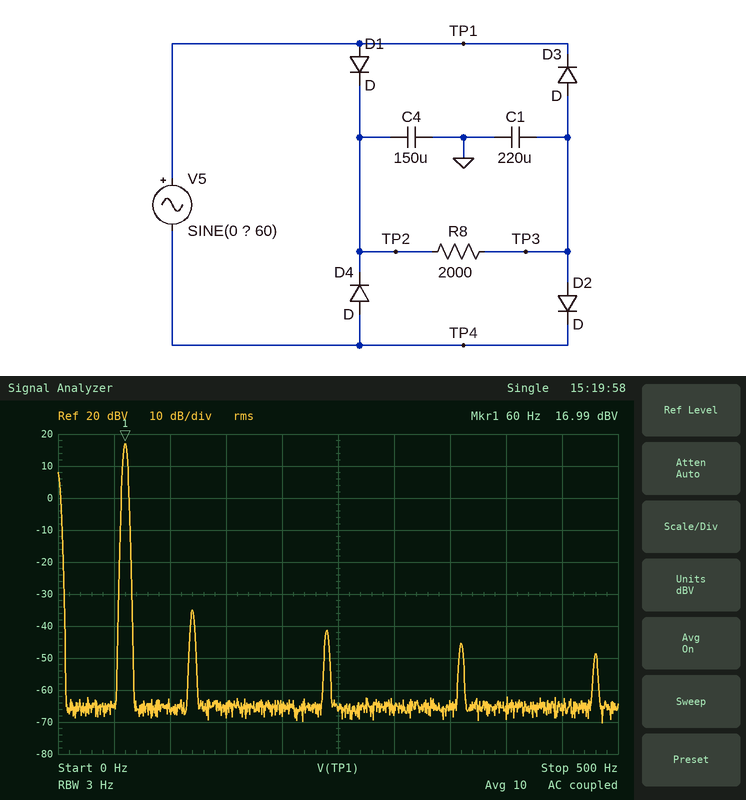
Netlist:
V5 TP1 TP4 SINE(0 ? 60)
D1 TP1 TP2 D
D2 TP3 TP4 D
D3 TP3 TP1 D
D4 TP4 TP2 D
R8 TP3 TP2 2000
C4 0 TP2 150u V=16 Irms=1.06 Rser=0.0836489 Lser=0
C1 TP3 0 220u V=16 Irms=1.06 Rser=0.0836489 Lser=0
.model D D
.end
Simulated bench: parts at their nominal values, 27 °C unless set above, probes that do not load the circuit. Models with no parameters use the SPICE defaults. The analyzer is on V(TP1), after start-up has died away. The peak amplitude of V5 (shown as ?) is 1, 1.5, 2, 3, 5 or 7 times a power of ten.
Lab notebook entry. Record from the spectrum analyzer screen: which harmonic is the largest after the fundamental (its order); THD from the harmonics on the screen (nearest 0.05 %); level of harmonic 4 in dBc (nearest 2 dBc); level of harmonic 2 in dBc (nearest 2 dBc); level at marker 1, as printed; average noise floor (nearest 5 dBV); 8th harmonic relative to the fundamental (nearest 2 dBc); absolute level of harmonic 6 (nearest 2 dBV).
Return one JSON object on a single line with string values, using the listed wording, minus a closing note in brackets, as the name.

{"which harmonic is the largest after the fundamental": "2", "THD from the harmonics on the screen": "0.30 %", "level of harmonic 4 in dBc": "-58 dBc", "level of harmonic 2 in dBc": "-52 dBc", "level at marker 1, as printed": "16.99 dBV", "average noise floor": "-65 dBV", "8th harmonic relative to the fundamental": "-66 dBc", "absolute level of harmonic 6": "-46 dBV"}
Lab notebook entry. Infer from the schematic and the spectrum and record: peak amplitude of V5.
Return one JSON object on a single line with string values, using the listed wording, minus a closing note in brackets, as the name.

{"peak amplitude of V5": "20 V"}
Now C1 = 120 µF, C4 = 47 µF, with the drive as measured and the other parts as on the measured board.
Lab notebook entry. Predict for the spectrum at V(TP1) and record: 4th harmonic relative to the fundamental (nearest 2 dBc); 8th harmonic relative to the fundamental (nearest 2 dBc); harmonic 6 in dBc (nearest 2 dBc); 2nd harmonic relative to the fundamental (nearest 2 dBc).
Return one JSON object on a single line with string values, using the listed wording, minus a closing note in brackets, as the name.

{"4th harmonic relative to the fundamental": "-44 dBc", "8th harmonic relative to the fundamental": "-52 dBc", "harmonic 6 in dBc": "-48 dBc", "2nd harmonic relative to the fundamental": "-36 dBc"}
